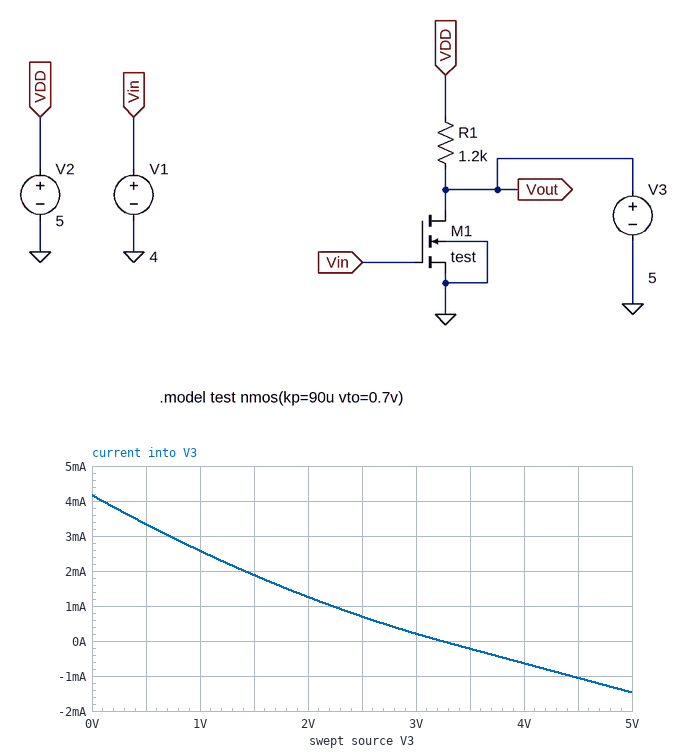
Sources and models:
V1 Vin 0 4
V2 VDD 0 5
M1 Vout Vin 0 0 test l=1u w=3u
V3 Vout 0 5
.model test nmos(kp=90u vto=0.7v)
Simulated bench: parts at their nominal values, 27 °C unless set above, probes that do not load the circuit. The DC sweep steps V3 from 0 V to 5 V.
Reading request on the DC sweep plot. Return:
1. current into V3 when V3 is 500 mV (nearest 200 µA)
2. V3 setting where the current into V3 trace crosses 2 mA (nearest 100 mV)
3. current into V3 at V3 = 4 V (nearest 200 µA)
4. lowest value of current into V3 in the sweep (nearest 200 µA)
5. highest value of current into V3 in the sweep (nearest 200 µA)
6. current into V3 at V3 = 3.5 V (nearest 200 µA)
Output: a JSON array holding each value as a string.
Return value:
["3.4 mA", "1.4 V", "-600 µA", "-1.4 mA", "4.2 mA", "-200 µA"]
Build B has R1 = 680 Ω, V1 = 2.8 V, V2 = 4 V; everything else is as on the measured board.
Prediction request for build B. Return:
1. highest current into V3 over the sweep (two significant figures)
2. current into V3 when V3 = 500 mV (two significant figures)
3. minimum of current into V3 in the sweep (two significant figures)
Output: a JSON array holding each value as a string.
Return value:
["5.9 mA", "4.9 mA", "-2.1 mA"]
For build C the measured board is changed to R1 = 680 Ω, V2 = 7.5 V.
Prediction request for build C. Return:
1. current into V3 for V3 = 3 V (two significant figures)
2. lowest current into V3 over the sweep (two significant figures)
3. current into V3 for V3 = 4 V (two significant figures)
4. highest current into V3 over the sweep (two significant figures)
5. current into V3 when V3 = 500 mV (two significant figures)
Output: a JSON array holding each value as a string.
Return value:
["5.2 mA", "2.2 mA", "3.7 mA", "11 mA", "9.9 mA"]
